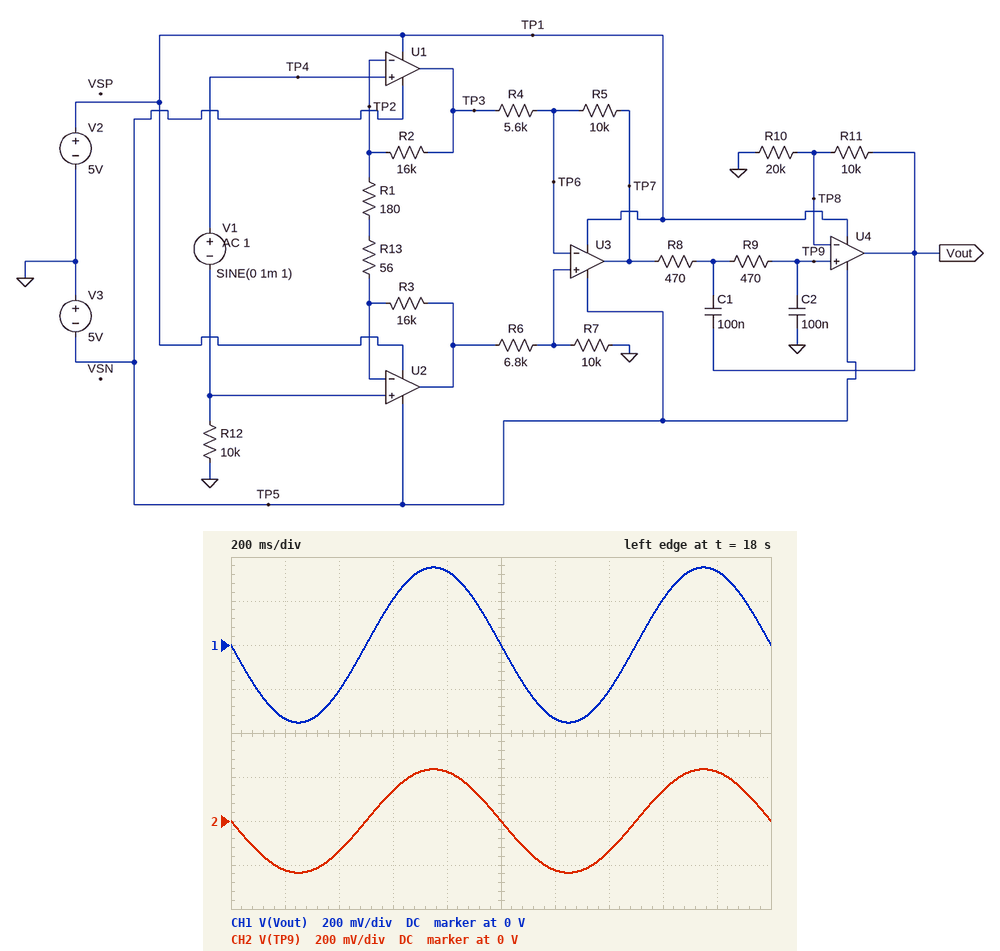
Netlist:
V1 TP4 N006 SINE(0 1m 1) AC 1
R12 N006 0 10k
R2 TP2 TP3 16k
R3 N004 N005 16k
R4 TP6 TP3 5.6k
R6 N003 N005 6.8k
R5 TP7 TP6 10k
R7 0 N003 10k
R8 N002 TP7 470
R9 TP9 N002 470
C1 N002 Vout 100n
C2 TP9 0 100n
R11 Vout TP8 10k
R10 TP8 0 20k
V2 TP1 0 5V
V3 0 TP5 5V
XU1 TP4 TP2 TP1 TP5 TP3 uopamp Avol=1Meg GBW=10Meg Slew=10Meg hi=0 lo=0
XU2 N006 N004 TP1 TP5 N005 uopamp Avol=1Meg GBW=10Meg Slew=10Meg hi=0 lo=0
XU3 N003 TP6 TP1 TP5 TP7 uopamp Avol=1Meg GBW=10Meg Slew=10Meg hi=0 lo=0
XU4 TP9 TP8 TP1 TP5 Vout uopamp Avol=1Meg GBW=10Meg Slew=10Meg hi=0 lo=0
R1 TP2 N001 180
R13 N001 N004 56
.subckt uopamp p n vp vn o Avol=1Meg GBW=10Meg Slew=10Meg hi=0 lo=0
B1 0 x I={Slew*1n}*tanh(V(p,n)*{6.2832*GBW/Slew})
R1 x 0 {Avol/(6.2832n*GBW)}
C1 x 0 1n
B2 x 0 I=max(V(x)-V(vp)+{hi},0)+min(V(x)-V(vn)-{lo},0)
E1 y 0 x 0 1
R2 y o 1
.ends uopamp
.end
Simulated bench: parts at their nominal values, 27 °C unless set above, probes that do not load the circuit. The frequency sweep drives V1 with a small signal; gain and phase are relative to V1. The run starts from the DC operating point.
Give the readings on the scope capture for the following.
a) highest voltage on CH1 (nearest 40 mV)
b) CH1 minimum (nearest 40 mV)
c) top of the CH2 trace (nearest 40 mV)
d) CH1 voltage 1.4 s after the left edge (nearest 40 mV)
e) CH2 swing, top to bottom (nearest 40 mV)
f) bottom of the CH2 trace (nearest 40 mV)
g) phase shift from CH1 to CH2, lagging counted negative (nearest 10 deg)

360 mV
-360 mV
240 mV
-200 mV
480 mV
-240 mV
0 deg
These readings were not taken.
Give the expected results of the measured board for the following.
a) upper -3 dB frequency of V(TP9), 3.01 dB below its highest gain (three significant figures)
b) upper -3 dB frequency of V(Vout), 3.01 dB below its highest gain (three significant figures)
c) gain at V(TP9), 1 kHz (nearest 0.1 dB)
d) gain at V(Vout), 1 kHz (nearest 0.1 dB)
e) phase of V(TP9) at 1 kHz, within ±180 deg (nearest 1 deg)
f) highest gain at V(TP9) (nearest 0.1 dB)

3.18 kHz
3.18 kHz
47.3 dB
50.8 dB
153 deg
47.4 dB
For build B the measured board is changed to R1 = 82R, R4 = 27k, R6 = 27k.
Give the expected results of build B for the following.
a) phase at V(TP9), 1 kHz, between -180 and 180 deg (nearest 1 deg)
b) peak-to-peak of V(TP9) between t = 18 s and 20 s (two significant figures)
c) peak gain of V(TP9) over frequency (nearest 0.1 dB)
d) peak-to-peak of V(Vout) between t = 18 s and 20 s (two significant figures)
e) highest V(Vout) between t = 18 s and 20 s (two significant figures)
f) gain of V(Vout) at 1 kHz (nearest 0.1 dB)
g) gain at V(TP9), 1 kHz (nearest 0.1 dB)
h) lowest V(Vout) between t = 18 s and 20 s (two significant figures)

153 deg
170 mV
38.7 dB
260 mV
130 mV
42.1 dB
38.6 dB
-130 mV
